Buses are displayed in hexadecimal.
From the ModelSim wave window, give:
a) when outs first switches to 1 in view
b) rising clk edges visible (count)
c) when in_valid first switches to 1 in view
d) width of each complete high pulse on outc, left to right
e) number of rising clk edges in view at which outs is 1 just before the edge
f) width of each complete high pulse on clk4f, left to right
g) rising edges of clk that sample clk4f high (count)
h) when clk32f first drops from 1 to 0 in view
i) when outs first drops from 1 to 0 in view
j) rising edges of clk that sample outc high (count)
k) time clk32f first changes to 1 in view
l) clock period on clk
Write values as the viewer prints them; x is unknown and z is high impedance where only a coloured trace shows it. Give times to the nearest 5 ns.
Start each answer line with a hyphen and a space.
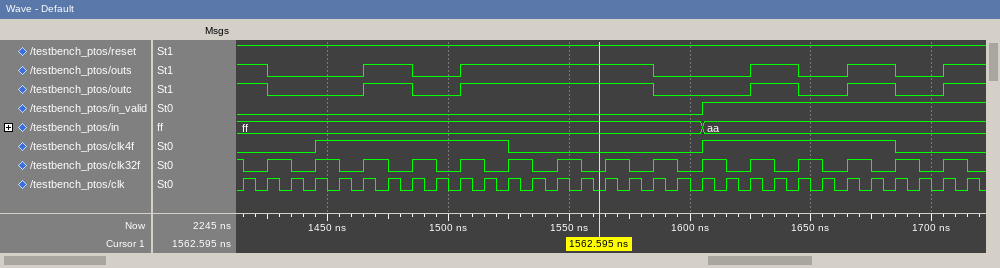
- 1465 ns
- 31
- 1605 ns
- 20 ns, 80 ns, 20 ns, 20 ns
- 17
- 80 ns, 80 ns
- 16
- 1415 ns
- 1425 ns
- 17
- 1425 ns
- 10 ns
